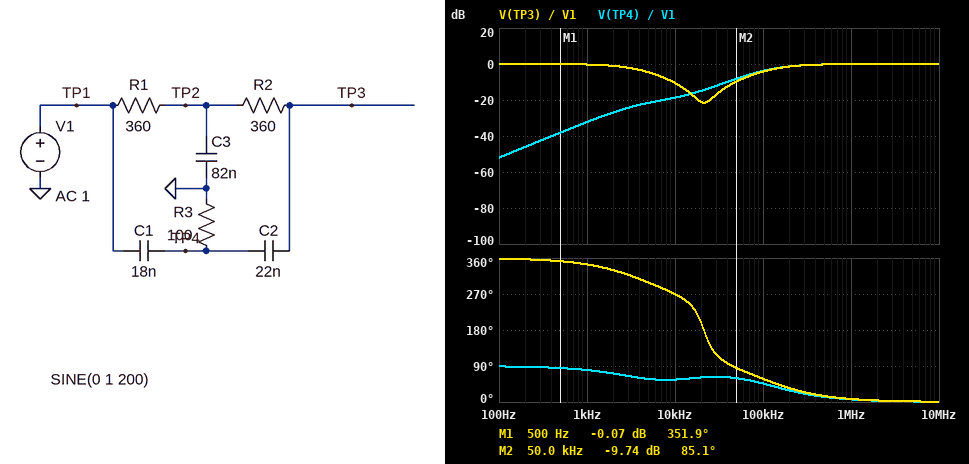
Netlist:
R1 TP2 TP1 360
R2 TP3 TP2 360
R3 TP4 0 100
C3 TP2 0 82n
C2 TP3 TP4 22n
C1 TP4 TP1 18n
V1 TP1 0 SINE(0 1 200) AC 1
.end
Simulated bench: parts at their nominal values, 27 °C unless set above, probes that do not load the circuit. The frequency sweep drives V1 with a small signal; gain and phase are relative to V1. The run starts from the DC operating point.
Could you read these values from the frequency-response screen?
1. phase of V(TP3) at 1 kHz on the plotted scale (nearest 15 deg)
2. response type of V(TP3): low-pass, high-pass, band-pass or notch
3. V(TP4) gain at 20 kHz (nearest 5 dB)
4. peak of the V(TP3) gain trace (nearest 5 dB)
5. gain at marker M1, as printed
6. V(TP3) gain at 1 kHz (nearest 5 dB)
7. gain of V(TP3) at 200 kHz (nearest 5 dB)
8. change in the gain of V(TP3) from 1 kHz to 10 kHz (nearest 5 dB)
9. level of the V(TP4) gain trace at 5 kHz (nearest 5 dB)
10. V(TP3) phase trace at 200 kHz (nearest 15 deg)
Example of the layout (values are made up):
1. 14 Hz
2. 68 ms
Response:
1. 345 deg
2. notch
3. -15 dB
4. 0 dB
5. -0.07 dB
6. 0 dB
7. 0 dB
8. -10 dB
9. -20 dB
10. 30 deg
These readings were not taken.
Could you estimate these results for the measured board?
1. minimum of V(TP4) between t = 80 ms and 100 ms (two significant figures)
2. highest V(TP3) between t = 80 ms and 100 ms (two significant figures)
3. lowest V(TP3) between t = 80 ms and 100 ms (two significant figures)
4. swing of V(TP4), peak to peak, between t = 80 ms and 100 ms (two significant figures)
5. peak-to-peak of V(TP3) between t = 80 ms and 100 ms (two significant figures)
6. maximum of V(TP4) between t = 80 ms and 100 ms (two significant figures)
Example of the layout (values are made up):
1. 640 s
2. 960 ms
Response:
1. -5.0 mV
2. 1.0 V
3. -1.0 V
4. 10 mV
5. 2.0 V
6. 5.0 mV
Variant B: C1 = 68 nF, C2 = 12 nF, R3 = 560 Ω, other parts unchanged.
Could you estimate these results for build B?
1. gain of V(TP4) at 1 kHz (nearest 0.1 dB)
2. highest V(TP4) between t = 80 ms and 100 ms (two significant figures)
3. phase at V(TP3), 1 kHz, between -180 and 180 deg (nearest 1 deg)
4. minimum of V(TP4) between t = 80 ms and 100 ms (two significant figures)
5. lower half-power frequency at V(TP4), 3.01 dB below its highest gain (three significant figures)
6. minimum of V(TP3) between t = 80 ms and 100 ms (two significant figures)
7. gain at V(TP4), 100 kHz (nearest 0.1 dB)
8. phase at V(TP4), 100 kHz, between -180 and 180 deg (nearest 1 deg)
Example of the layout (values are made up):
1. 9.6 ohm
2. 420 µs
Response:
1. -11.4 dB
2. 56 mV
3. -13 deg
4. -56 mV
5. 4.24 kHz
6. -1.0 V
7. -0.3 dB
8. 5 deg
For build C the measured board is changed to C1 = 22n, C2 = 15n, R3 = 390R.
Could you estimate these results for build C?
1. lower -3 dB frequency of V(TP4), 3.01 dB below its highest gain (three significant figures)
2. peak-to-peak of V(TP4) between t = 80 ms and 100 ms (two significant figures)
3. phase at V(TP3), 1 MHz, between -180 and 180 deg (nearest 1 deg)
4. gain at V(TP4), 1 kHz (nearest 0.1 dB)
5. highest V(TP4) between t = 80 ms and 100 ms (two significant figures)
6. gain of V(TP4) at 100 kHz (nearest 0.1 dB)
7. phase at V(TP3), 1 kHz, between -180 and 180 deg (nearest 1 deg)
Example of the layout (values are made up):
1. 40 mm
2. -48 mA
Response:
1. 47.1 kHz
2. 36 mV
3. 4 deg
4. -21.1 dB
5. 18 mV
6. -1.1 dB
7. -14 deg
